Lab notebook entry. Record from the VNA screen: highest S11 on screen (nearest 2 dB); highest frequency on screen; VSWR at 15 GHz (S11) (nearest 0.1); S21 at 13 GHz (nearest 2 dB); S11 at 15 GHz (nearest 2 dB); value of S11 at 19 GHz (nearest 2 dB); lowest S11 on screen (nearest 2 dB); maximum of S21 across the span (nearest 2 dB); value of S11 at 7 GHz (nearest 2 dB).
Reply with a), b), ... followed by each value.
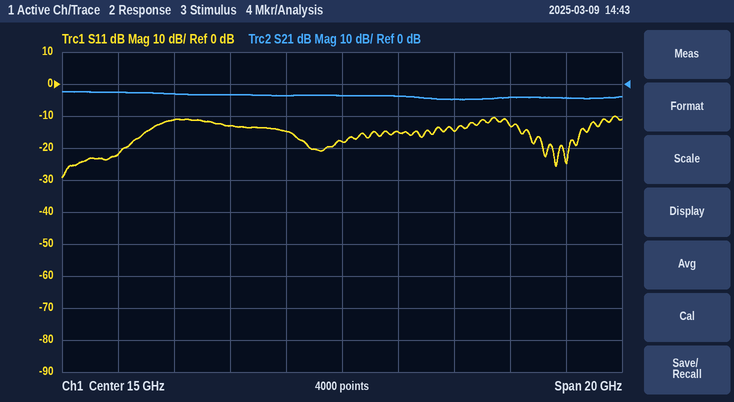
a) -10 dB
b) 25 GHz
c) 1.3
d) -4 dB
e) -18 dB
f) -14 dB
g) -30 dB
h) -2 dB
i) -22 dB
